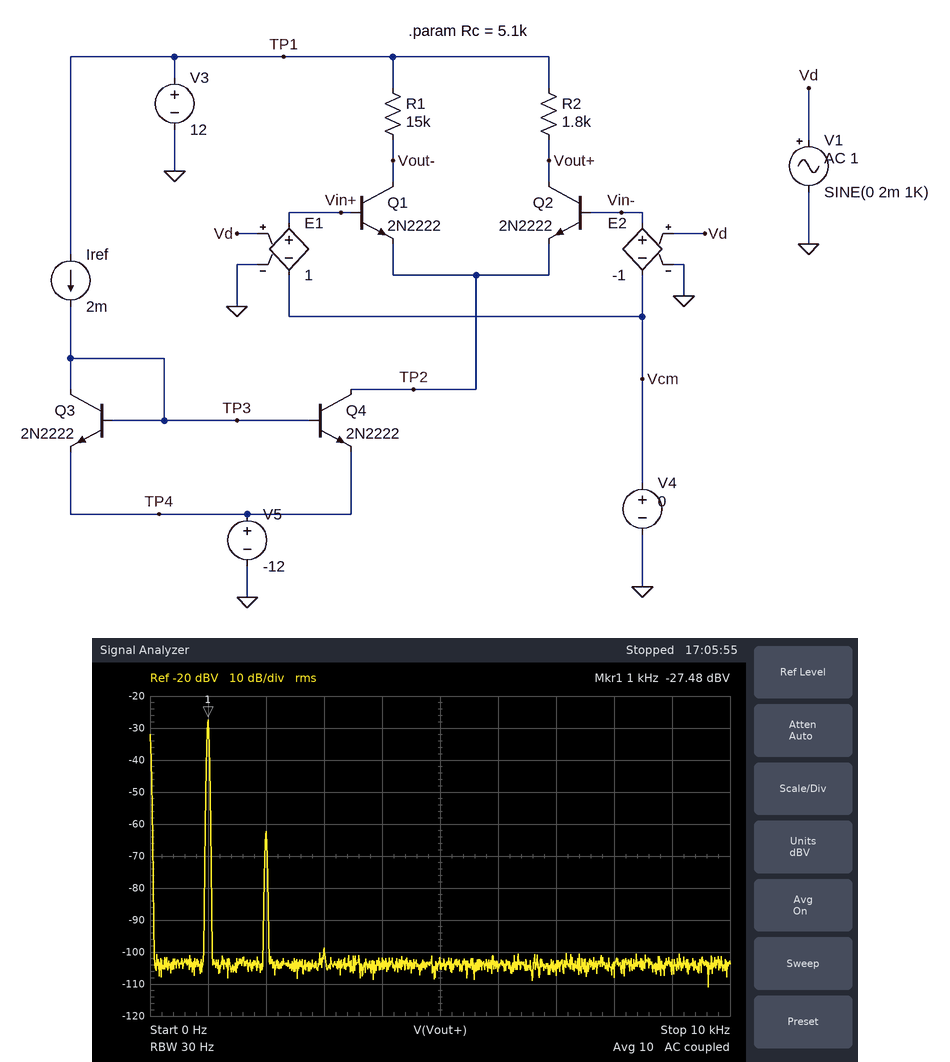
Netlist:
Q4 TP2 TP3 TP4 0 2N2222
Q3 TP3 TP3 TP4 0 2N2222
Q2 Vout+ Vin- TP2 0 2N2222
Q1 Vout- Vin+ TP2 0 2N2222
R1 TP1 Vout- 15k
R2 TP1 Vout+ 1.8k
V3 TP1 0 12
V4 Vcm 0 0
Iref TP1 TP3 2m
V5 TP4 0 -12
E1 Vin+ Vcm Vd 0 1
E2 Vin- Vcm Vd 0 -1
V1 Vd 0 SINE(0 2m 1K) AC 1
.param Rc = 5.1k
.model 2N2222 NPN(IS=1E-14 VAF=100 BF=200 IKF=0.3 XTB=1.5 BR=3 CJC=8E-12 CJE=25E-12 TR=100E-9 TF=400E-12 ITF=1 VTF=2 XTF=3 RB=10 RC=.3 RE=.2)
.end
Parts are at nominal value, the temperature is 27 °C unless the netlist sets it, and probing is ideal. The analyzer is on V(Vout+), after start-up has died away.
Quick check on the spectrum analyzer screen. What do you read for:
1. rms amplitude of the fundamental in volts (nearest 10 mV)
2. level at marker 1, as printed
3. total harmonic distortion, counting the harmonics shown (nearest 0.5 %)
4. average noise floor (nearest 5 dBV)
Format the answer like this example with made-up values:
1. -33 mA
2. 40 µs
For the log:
1. 40 mV
2. -27.48 dBV
3. 2.0 %
4. -105 dBV
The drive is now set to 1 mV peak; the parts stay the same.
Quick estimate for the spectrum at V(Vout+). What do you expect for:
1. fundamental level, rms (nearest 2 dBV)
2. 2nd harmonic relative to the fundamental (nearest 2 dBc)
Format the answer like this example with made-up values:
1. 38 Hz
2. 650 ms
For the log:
1. -34 dBV
2. -40 dBc
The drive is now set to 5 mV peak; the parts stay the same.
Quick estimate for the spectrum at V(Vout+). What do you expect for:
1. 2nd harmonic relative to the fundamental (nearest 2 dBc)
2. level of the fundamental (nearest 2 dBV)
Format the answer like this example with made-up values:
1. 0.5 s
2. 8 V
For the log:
1. -28 dBc
2. -20 dBV
